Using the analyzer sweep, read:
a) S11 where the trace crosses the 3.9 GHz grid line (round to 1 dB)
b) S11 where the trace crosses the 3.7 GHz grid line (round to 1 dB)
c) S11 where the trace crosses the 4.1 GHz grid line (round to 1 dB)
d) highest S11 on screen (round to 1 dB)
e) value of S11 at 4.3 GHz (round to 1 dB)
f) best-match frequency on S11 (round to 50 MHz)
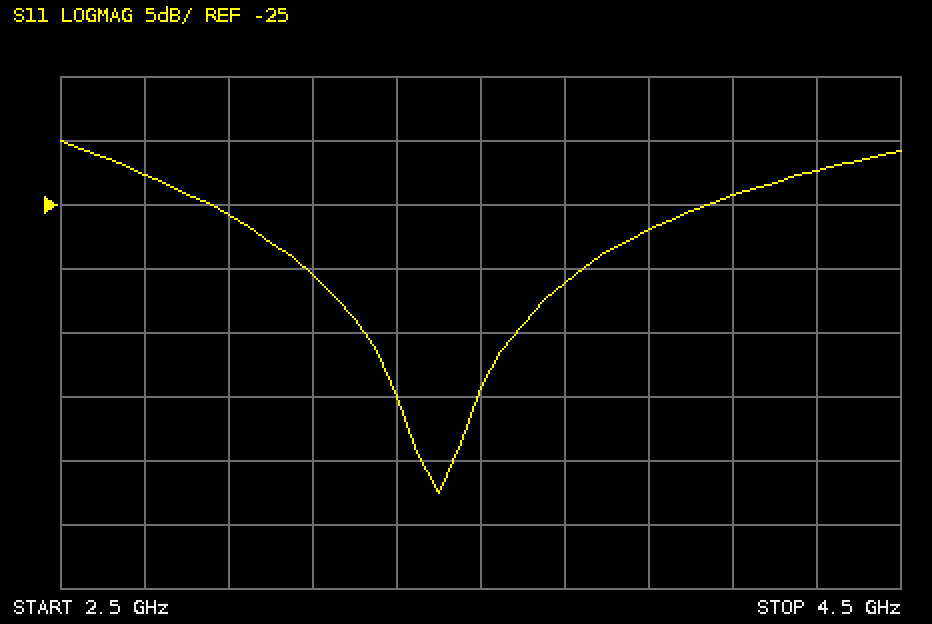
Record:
-27 dB
-31 dB
-24 dB
-20 dB
-22 dB
3.40 GHz
